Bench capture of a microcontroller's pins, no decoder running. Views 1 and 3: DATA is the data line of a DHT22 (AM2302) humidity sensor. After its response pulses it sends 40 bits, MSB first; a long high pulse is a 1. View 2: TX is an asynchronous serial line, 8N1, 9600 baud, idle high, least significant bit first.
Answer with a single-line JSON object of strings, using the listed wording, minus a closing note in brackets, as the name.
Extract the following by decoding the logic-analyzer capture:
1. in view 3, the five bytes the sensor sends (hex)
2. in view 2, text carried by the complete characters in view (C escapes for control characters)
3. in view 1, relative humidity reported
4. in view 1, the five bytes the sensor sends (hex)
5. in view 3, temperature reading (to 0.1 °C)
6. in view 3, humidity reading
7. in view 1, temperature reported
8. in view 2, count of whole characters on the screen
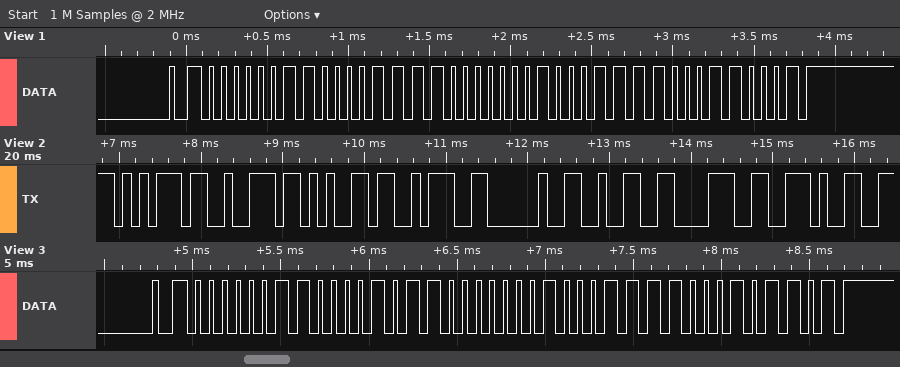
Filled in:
{"in view 3, the five bytes the sensor sends": "03 0B 01 1E 2D", "in view 2, text carried by the complete characters in view": "\"ure: 28.\"", "in view 1, relative humidity reported": "78.3 %", "in view 1, the five bytes the sensor sends": "03 0F 01 1E 31", "in view 3, temperature reading": "28.6 °C", "in view 3, humidity reading": "77.9 %", "in view 1, temperature reported": "28.6 °C", "in view 2, count of whole characters on the screen": "8"}
